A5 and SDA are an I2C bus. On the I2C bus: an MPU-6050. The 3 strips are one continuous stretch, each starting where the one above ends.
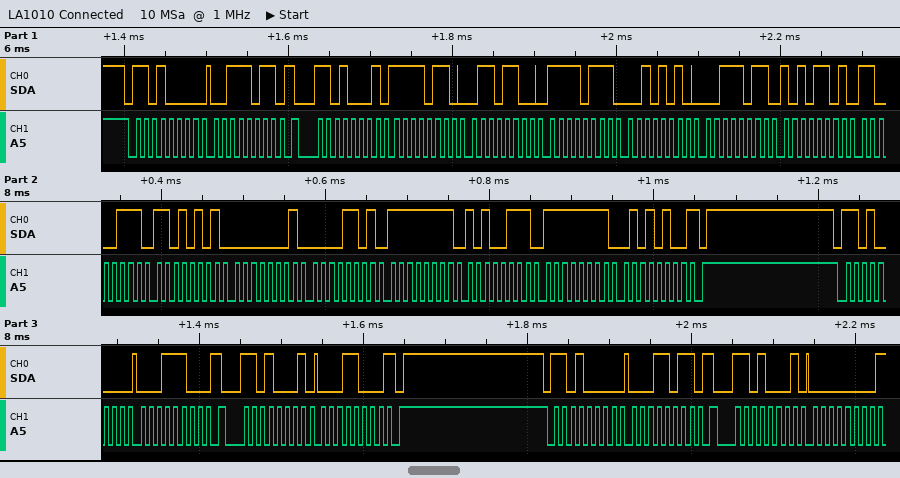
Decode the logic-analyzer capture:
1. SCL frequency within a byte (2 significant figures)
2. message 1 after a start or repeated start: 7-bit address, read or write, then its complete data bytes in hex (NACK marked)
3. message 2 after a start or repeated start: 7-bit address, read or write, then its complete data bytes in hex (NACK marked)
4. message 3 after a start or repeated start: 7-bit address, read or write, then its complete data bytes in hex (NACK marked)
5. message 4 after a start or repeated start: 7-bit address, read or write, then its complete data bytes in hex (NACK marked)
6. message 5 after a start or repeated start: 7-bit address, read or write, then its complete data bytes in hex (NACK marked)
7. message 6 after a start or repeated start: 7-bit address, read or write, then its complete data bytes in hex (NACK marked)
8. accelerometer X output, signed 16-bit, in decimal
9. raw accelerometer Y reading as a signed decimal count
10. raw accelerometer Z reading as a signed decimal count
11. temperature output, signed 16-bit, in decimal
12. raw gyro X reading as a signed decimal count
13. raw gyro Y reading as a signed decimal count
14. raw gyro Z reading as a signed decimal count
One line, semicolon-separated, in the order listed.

100 kHz; 0x68 write: 3B; 0x68 read: F6 6C F7 2A 3B AD C7 D5 01 0D FF A7 FF 54 NACK; 0x68 write: 1C; 0x68 read: 18 NACK; 0x68 write: 1B; 0x68 read: 00 NACK; -2452; -2262; 15277; -14379; 269; -89; -172
